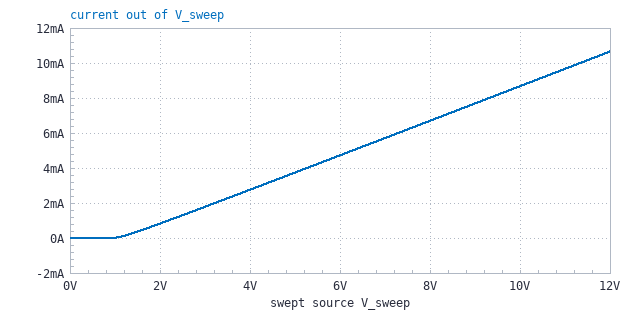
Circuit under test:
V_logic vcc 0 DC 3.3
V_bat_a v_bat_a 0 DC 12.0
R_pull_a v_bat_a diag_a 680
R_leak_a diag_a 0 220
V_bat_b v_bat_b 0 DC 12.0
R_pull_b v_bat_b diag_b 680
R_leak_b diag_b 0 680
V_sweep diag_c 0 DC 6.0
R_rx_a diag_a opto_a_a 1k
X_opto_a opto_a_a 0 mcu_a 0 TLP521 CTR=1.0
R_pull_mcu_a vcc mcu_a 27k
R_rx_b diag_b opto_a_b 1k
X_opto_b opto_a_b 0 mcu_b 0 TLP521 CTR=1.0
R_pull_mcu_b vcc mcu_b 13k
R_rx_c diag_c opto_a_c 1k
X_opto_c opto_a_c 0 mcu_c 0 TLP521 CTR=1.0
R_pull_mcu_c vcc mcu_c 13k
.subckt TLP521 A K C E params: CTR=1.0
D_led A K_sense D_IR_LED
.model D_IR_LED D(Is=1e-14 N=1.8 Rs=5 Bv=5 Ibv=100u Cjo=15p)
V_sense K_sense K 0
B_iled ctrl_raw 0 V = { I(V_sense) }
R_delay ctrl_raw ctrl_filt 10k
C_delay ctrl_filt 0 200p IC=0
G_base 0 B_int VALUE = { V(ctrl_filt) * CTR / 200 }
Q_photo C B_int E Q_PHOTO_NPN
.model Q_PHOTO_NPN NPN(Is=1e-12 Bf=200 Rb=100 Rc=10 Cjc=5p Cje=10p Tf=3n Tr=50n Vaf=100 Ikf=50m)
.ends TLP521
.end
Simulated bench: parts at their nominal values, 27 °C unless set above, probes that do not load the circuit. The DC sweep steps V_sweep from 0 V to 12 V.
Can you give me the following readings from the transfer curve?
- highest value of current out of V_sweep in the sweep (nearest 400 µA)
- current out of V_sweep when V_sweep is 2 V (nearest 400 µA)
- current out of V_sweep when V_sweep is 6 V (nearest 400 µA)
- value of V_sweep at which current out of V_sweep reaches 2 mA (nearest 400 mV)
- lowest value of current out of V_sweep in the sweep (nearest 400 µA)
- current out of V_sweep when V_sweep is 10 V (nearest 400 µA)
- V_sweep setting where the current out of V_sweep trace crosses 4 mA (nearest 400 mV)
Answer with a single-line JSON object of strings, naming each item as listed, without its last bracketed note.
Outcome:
{"highest value of current out of V_sweep in the sweep": "10.8 mA", "current out of V_sweep when V_sweep is 2 V": "800 µA", "current out of V_sweep when V_sweep is 6 V": "4.8 mA", "value of V_sweep at which current out of V_sweep reaches 2 mA": "3.2 V", "lowest value of current out of V_sweep in the sweep": "0 A", "current out of V_sweep when V_sweep is 10 V": "8.8 mA", "V_sweep setting where the current out of V_sweep trace crosses 4 mA": "5.2 V"}
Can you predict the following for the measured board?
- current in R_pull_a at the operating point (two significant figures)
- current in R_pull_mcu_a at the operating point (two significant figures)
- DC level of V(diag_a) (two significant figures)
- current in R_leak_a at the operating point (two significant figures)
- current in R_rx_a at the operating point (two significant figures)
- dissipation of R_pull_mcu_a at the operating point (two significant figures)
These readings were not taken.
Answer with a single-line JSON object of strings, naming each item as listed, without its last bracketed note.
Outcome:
{"current in R_pull_a at the operating point": "14 mA", "current in R_pull_mcu_a at the operating point": "120 µA", "DC level of V(diag_a)": "2.7 V", "current in R_leak_a at the operating point": "12 mA", "current in R_rx_a at the operating point": "1.5 mA", "dissipation of R_pull_mcu_a at the operating point": "380 µW"}
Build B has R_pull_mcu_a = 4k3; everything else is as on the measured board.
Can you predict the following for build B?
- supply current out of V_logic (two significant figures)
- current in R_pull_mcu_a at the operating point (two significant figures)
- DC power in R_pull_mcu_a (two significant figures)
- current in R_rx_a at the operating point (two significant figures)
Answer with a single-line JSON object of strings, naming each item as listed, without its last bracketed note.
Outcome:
{"supply current out of V_logic": "1.2 mA", "current in R_pull_mcu_a at the operating point": "730 µA", "DC power in R_pull_mcu_a": "2.3 mW", "current in R_rx_a at the operating point": "1.5 mA"}
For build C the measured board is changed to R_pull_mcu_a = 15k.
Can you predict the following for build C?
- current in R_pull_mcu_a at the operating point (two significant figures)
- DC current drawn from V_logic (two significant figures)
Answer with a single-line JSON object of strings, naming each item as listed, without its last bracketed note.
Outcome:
{"current in R_pull_mcu_a at the operating point": "210 µA", "DC current drawn from V_logic": "710 µA"}
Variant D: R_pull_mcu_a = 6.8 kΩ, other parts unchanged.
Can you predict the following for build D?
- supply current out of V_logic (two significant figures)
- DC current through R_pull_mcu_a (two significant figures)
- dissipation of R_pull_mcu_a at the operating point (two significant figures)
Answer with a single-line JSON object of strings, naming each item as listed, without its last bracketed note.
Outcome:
{"supply current out of V_logic": "960 µA", "DC current through R_pull_mcu_a": "470 µA", "dissipation of R_pull_mcu_a at the operating point": "1.5 mW"}
